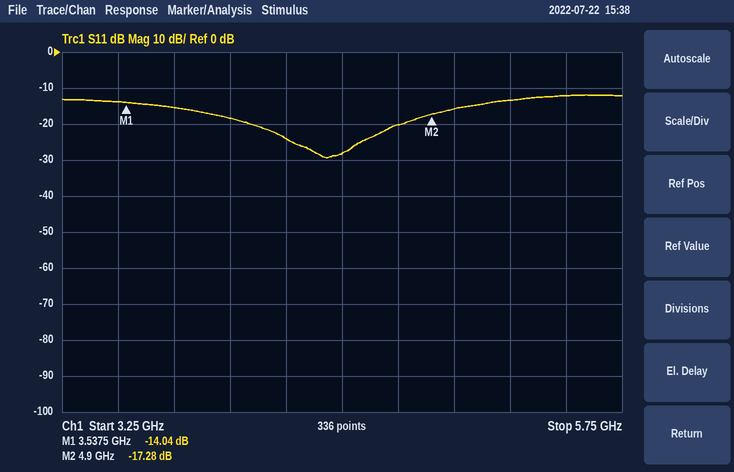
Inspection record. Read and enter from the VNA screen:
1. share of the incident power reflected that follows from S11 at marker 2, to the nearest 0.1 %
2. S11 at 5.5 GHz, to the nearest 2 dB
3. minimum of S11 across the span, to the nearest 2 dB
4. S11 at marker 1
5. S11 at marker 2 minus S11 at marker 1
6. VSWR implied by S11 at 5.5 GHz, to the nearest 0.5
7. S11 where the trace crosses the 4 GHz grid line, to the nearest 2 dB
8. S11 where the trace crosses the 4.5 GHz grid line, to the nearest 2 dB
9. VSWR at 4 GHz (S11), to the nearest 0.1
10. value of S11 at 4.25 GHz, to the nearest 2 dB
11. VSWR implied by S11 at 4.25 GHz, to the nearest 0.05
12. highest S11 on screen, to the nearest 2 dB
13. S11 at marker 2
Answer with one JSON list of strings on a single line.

["1.9 %", "-12 dB", "-30 dB", "-14.04 dB", "-3.24 dB", "1.5", "-18 dB", "-28 dB", "1.3", "-24 dB", "1.15", "-12 dB", "-17.28 dB"]
